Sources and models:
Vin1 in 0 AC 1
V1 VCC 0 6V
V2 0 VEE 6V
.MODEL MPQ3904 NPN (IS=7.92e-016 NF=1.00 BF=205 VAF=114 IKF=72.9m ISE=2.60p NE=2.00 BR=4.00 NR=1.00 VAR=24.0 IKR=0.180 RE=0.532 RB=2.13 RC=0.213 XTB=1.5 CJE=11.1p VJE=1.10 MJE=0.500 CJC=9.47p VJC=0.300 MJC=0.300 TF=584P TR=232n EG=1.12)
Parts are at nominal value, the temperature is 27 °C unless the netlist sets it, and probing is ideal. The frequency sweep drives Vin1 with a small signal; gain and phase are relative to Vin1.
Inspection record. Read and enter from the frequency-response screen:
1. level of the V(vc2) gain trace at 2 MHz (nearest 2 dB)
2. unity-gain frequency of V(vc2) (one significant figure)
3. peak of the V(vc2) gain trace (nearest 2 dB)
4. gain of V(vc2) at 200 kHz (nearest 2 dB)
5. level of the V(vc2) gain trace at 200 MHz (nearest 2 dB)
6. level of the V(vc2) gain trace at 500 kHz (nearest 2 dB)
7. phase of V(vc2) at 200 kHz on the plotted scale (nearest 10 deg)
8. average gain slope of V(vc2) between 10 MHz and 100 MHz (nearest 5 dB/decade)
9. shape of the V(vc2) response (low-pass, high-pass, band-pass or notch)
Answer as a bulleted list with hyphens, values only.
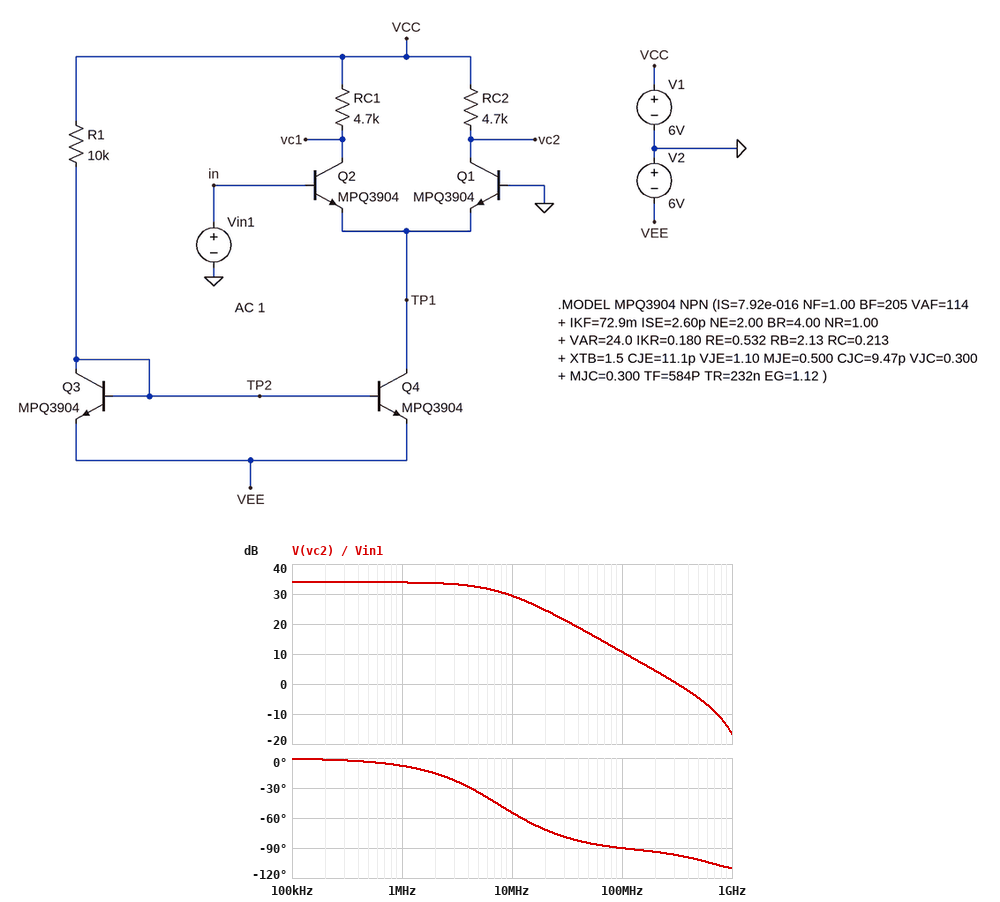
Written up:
- 34 dB
- 300 MHz
- 34 dB
- 34 dB
- 4 dB
- 34 dB
- 0 deg
- -20 dB/decade
- low-pass
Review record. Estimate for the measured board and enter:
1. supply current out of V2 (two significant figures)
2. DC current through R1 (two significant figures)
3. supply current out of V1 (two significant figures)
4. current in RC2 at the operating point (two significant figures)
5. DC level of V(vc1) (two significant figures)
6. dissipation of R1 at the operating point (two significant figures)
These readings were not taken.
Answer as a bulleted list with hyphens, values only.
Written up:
- 2.3 mA
- 1.1 mA
- 2.3 mA
- 570 µA
- 3.3 V
- 13 mW
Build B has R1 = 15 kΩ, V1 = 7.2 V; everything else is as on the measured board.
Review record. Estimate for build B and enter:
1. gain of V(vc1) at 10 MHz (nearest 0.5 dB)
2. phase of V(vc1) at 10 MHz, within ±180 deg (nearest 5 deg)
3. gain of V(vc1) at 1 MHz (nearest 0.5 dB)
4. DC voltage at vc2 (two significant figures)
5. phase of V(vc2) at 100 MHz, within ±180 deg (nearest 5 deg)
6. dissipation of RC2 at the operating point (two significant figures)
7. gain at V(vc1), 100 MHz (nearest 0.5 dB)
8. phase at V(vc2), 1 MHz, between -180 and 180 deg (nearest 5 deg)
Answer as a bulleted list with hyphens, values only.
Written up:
- 27.5 dB
- 130 deg
- 31.5 dB
- 5.2 V
- -90 deg
- 840 µW
- 11.0 dB
- -5 deg
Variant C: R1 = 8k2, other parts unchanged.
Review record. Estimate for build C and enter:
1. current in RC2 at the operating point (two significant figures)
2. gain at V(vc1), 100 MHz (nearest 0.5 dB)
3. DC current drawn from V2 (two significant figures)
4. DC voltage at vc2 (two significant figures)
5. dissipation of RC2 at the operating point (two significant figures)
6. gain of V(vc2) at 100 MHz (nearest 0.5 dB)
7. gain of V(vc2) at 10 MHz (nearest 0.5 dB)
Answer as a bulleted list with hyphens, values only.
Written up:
- 700 µA
- 13.0 dB
- 2.8 mA
- 2.7 V
- 2.3 mW
- 12.0 dB
- 30.5 dB
